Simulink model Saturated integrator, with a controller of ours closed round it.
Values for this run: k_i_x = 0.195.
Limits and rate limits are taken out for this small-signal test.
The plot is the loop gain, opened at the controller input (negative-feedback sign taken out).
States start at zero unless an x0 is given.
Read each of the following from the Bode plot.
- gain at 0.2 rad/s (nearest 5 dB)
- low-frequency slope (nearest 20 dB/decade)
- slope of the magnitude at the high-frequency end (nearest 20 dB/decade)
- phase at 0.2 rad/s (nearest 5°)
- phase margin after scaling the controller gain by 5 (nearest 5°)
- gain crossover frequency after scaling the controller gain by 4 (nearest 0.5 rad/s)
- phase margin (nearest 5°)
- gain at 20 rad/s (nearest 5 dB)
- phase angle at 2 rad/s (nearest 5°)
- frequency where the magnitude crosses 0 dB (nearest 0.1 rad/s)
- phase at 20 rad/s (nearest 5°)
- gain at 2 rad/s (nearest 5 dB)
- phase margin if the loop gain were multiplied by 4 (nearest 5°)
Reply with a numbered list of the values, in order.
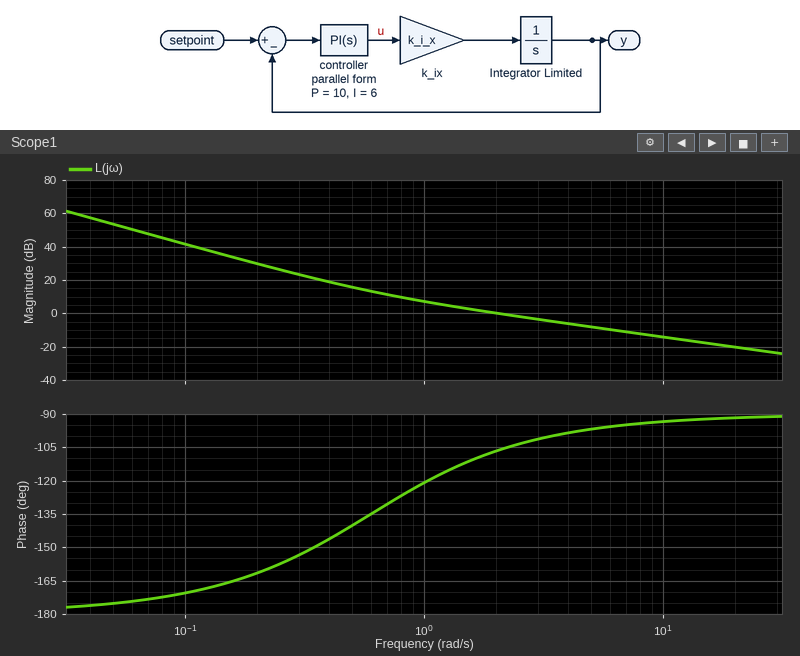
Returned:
1. 30 dB
2. -40 dB/decade
3. -20 dB/decade
4. -160°
5. 85°
6. 8.0 rad/s
7. 75°
8. -20 dB
9. -105°
10. 2.0 rad/s
11. -90°
12. 0 dB
13. 85°
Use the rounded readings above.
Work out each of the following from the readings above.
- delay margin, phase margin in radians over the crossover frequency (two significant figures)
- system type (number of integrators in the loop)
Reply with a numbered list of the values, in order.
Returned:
1. 0.65 s
2. 2
